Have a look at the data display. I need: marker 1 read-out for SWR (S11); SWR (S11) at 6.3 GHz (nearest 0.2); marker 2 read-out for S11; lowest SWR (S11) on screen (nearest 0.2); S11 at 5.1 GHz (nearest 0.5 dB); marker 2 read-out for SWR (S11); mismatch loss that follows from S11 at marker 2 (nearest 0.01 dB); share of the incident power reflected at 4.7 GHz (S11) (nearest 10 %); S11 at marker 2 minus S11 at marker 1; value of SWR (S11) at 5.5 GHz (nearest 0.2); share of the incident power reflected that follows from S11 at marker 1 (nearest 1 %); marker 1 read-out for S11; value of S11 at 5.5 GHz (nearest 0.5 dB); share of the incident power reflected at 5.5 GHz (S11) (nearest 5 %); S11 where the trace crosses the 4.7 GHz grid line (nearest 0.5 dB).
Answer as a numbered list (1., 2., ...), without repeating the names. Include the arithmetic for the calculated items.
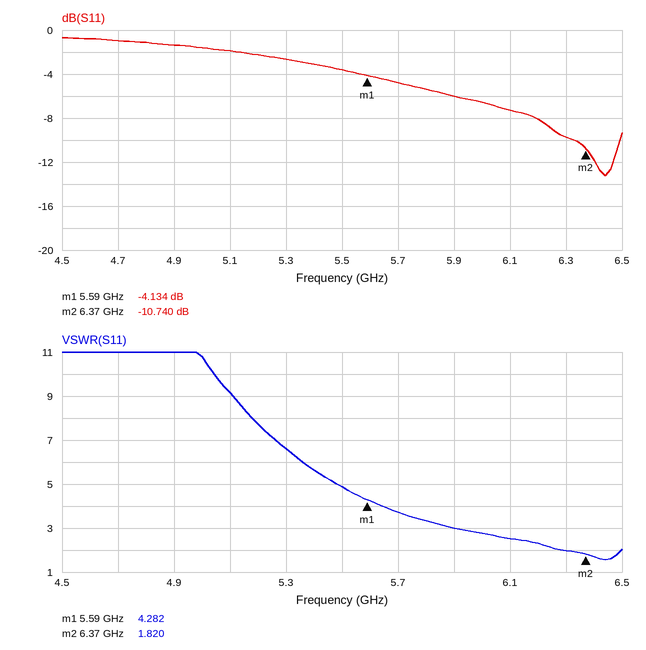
1. 4.282
2. 2.0
3. -10.740 dB
4. 1.6
5. -2.0 dB
6. 1.820
7. −10 log10(1 − 10^(-10.74/10)) ≈ 0.38 dB
8. 10^(-1/10) ≈ 79.4 %, so 80 % to the nearest 10 %
9. -10.74 − (-4.134) = -6.606 dB
10. 4.8
11. 10^(-4.134/10) ≈ 39 %
12. -4.134 dB
13. -3.5 dB
14. 10^(-3.5/10) ≈ 45 %
15. -1.0 dB
